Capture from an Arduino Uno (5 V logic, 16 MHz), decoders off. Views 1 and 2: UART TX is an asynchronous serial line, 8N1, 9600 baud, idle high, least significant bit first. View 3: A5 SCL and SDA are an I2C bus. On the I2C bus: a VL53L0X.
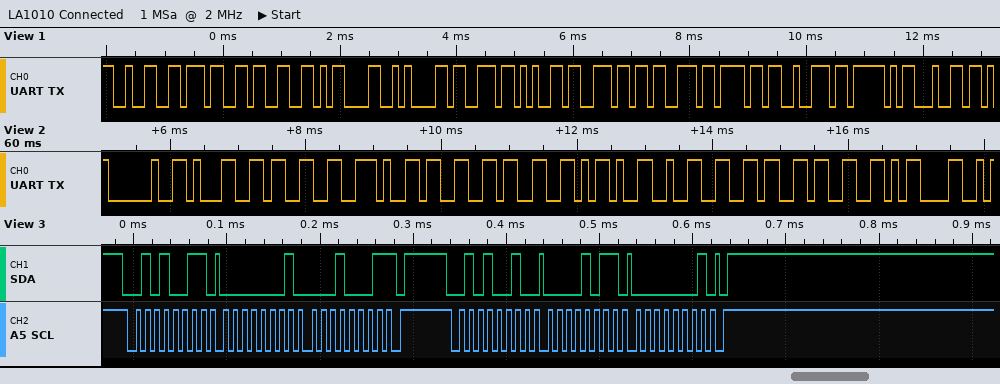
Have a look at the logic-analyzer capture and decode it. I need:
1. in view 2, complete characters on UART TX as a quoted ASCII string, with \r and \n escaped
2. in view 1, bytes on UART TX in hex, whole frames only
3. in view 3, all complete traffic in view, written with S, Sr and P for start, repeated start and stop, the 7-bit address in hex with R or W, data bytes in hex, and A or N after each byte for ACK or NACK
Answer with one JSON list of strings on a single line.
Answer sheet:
["\" 13.33-263\\r\"", "32 37 33 0D 0A 73 65 6E 73 6F 72 5F 64", "S 29R A 01 A 11 N P S 29W A 0B A 01 A P"]
